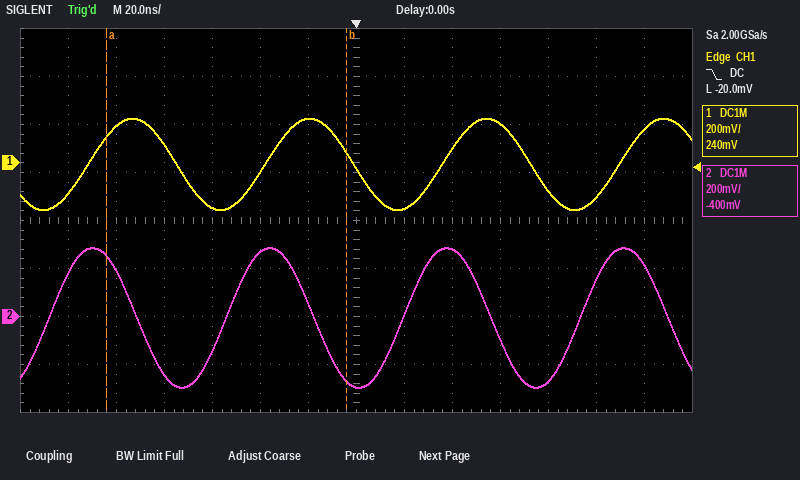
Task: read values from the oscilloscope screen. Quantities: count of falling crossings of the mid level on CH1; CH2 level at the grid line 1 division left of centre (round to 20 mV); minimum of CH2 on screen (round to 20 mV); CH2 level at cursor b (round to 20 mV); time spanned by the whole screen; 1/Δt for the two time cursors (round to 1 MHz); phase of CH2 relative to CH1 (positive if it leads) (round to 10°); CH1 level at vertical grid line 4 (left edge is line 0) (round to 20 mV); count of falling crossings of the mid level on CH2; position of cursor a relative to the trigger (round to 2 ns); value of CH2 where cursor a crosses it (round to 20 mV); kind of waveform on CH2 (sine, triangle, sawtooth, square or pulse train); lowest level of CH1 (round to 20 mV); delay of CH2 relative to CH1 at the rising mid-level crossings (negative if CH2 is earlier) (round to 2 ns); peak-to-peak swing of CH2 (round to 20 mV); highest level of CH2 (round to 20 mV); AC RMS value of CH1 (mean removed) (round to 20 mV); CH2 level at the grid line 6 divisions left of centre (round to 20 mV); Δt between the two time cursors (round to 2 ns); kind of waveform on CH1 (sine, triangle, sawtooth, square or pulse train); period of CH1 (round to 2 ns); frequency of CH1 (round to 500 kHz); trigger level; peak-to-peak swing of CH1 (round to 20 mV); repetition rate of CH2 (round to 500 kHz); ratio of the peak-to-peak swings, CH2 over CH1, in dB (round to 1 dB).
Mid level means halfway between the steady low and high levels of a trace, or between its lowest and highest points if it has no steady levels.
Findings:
3
60 mV
-300 mV
-260 mV
280 ns
10 MHz
+80°
-180 mV
4
-104 ns
260 mV
sine
-200 mV
-16 ns
580 mV
280 mV
140 mV
180 mV
100 ns
sine
74 ns
13.5 MHz
-20.0 mV
380 mV
13.5 MHz
4 dB
